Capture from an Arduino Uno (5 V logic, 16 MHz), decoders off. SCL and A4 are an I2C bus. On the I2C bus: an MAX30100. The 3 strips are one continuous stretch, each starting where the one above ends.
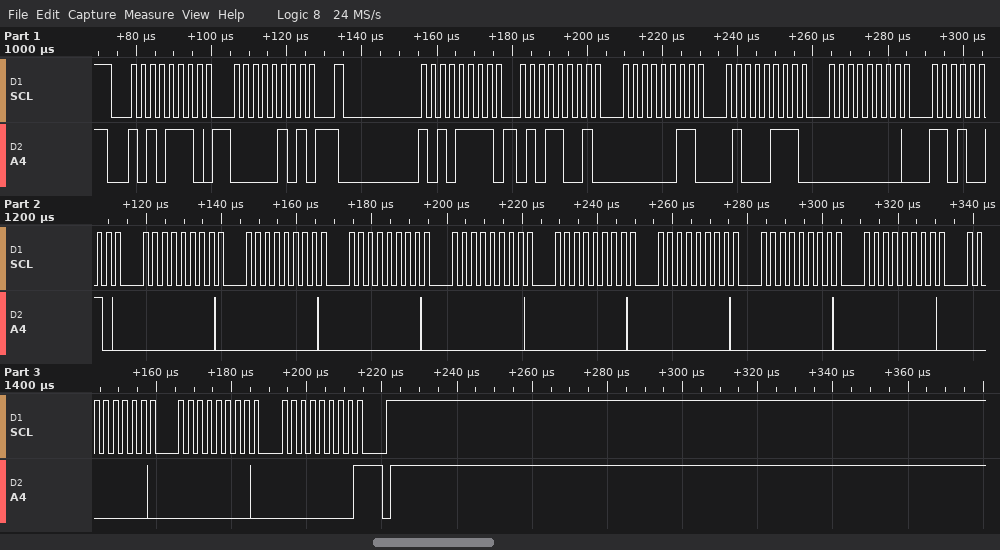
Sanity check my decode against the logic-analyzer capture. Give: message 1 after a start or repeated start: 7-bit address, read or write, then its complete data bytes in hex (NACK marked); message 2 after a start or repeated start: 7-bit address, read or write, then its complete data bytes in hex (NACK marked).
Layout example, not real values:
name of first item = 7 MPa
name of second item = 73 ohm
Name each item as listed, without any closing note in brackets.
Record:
message 1 after a start or repeated start: 7-bit address, read or write, then its complete data bytes in hex = 0x57 write: 05
message 2 after a start or repeated start: 7-bit address, read or write, then its complete data bytes in hex = 0x57 read: 59 03 47 00 D2 00 00 00 00 00 00 00 00 00 00 00 NACK
